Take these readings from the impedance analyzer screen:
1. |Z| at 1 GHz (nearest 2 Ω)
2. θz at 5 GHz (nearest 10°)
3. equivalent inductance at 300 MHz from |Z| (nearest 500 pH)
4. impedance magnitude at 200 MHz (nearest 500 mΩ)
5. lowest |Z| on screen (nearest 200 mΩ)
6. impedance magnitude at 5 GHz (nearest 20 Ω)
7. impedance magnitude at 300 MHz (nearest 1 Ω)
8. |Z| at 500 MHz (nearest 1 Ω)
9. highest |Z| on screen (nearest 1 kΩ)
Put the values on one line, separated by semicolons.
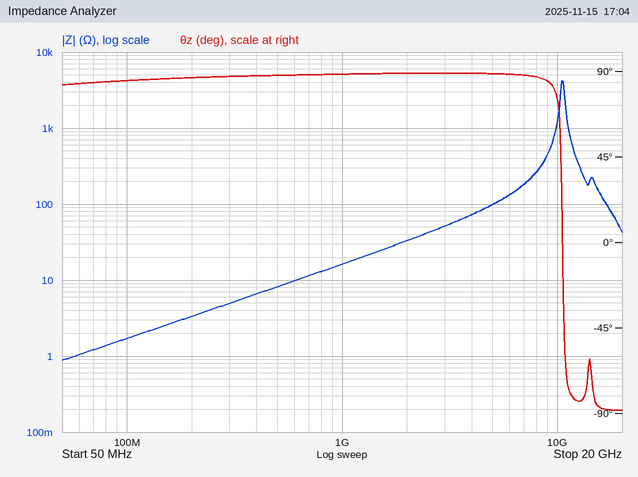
16 Ω; 90°; 2.5 nH; 3.5 Ω; 800 mΩ; 100 Ω; 5 Ω; 8 Ω; 4 kΩ
